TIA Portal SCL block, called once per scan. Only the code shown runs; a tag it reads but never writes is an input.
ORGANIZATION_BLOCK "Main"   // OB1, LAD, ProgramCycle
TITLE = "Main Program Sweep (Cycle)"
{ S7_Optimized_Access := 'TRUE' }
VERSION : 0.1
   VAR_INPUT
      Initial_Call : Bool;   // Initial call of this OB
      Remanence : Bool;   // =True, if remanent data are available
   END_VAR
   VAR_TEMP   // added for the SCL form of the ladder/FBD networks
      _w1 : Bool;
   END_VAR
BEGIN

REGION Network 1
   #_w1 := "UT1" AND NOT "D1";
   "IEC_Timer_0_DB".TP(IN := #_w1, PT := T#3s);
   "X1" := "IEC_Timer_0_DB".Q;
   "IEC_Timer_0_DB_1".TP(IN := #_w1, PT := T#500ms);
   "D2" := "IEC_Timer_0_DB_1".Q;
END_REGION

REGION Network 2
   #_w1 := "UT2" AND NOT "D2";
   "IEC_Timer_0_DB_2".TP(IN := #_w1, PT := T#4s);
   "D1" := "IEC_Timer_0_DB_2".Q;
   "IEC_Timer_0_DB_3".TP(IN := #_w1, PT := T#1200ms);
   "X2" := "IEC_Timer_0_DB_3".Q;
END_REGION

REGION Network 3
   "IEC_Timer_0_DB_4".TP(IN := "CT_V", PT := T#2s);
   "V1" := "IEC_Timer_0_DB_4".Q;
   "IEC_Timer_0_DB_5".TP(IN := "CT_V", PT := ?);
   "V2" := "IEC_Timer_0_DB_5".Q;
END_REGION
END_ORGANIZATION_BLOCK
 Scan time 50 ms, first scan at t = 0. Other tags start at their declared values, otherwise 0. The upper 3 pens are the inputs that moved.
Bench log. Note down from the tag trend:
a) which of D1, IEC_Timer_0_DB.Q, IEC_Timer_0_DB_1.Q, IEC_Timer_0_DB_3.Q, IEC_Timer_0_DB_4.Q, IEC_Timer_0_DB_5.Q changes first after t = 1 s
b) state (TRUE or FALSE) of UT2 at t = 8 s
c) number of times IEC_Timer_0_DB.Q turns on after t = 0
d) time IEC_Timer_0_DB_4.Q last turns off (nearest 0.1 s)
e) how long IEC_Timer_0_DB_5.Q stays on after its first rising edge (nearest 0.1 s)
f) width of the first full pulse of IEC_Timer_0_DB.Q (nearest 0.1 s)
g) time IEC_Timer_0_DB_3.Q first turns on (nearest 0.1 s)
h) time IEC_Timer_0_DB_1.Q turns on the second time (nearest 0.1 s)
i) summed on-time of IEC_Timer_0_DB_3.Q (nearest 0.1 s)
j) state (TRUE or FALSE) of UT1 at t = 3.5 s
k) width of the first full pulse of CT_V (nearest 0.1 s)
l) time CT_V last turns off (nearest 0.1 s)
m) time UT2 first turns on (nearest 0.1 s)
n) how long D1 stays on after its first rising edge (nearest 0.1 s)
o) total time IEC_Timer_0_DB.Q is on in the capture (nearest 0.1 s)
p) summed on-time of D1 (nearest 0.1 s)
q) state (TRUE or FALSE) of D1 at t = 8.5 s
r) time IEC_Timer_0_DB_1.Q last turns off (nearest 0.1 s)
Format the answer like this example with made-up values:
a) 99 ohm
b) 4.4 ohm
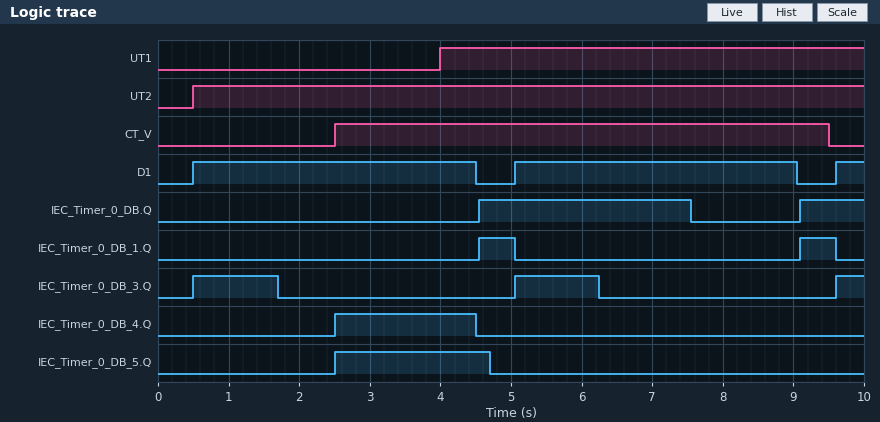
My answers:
a) IEC_Timer_0_DB_3.Q
b) TRUE
c) 2
d) 4.5 s
e) 2.2 s
f) 3.0 s
g) 0.5 s
h) 9.1 s
i) 2.8 s
j) FALSE
k) 7.0 s
l) 9.5 s
m) 0.5 s
n) 4.0 s
o) 3.9 s
p) 8.4 s
q) TRUE
r) 9.6 s
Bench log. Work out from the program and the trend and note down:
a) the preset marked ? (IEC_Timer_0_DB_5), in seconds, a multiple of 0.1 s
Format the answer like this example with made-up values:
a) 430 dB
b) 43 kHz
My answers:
a) 2.2 s
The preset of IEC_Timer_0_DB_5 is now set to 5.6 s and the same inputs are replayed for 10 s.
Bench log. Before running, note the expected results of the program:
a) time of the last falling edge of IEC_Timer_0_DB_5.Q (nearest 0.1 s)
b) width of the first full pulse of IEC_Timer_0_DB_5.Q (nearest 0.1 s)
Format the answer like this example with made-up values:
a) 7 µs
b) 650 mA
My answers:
a) 8.1 s
b) 5.6 s
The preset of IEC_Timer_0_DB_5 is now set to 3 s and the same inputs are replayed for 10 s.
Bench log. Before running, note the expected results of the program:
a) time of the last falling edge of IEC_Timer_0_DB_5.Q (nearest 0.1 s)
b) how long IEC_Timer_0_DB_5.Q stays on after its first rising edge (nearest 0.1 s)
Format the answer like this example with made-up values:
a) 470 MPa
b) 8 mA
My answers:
a) 5.5 s
b) 3.0 s
